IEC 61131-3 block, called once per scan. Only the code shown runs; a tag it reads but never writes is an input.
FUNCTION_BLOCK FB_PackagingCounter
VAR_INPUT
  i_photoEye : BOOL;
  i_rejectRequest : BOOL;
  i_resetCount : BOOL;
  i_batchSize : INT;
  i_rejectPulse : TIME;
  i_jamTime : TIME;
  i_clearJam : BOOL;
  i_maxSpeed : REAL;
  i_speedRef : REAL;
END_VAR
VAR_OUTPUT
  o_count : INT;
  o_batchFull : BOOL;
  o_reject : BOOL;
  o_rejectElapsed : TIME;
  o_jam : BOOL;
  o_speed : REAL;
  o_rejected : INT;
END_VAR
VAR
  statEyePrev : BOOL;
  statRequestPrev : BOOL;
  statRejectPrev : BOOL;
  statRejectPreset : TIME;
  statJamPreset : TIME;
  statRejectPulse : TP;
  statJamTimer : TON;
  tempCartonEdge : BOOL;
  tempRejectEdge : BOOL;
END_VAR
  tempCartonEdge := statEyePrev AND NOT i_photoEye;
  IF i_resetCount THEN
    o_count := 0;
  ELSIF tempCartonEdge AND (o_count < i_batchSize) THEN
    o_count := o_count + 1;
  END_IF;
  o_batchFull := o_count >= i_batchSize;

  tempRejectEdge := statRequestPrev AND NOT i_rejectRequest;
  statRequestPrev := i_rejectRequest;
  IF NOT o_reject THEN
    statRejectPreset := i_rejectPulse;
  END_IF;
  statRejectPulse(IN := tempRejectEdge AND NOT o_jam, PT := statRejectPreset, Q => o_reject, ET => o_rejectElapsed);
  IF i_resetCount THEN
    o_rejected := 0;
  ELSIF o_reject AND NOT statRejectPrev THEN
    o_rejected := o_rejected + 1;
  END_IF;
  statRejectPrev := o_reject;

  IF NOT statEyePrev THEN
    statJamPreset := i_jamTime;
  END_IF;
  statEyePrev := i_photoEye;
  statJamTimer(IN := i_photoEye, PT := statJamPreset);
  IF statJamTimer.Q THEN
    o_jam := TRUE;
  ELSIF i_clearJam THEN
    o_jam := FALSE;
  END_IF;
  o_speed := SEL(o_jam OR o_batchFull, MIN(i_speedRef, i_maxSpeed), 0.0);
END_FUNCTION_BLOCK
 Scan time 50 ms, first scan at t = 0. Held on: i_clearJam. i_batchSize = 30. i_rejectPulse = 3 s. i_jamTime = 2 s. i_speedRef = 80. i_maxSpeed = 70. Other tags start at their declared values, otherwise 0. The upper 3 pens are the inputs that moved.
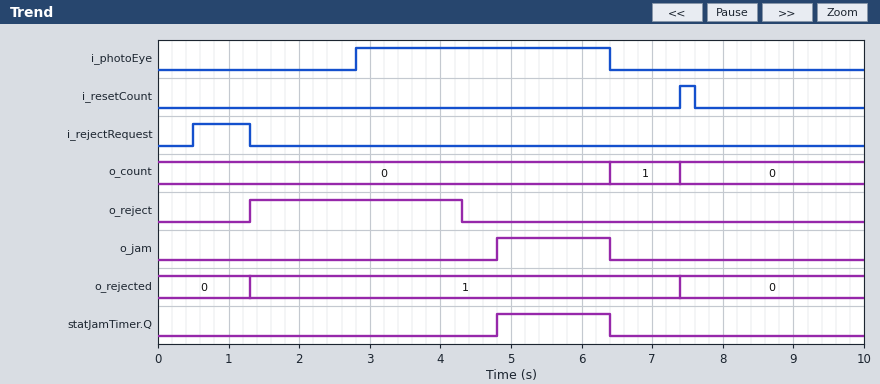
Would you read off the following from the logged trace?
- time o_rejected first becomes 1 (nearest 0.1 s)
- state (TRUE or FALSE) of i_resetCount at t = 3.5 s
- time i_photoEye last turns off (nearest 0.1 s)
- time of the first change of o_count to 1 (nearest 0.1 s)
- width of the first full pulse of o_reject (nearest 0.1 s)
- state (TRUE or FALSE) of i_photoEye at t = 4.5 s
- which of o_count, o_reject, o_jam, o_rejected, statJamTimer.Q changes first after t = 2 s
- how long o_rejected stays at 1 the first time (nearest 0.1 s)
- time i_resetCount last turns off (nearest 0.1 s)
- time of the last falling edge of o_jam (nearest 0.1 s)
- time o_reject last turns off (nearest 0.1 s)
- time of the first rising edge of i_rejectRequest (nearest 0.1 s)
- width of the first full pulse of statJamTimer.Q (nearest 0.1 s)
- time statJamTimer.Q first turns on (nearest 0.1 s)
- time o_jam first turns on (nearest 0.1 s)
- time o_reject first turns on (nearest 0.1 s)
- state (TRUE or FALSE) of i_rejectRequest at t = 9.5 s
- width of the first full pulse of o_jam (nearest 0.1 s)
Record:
1.3 s
FALSE
6.4 s
6.4 s
3.0 s
TRUE
o_reject
6.1 s
7.6 s
6.4 s
4.3 s
0.5 s
1.6 s
4.8 s
4.8 s
1.3 s
FALSE
1.6 s
